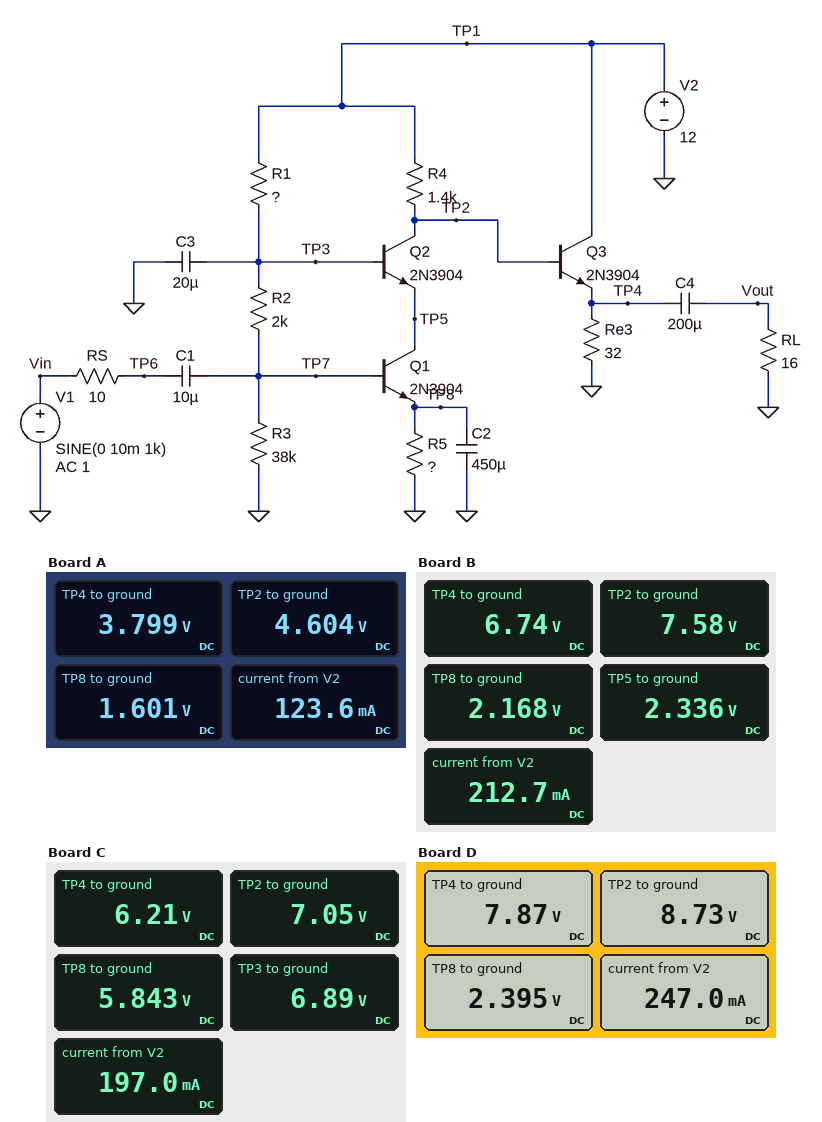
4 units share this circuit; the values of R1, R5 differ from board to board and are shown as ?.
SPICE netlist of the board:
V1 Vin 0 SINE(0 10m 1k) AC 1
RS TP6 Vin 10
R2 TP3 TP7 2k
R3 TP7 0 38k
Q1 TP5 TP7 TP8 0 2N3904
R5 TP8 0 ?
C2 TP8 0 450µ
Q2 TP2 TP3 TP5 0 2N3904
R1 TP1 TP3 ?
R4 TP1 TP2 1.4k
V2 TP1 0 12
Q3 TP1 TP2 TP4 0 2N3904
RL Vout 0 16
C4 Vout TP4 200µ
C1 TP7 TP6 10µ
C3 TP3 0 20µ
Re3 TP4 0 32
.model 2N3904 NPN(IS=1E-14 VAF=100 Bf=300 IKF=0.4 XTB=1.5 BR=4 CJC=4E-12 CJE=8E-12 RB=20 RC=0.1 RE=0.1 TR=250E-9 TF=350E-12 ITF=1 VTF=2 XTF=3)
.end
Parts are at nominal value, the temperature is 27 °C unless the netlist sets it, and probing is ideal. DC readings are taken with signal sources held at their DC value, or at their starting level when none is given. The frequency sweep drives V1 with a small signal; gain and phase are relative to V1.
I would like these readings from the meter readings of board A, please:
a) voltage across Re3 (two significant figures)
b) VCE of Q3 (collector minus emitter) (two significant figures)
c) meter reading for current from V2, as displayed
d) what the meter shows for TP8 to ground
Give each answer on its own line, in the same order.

3.8 V
8.2 V
123.6 mA
1.601 V
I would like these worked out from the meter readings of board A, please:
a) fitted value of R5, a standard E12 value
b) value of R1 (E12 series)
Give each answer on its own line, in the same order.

330 Ω
100 kΩ
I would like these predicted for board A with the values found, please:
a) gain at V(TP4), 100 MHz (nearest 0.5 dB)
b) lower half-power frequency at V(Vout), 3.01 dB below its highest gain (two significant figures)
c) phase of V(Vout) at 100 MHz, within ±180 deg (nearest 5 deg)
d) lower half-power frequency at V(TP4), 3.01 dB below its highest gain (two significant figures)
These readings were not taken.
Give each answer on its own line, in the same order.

1.0 dB
91 Hz
-35 deg
66 Hz
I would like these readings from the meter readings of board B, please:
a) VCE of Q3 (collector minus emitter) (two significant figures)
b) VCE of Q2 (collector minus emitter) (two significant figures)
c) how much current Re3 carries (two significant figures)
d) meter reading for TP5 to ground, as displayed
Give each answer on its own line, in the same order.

5.3 V
5.2 V
210 mA
2.336 V
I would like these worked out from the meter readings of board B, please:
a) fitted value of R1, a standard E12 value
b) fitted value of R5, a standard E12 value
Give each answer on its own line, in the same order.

100 kΩ
1 kΩ
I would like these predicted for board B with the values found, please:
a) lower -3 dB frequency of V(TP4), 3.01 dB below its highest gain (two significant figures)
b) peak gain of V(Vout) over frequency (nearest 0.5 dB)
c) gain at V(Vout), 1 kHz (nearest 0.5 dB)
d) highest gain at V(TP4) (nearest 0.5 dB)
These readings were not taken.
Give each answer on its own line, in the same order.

26 Hz
35.5 dB
35.5 dB
35.5 dB
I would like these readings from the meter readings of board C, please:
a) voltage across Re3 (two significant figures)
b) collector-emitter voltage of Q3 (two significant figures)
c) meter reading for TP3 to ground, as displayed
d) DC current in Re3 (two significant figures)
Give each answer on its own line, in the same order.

6.2 V
5.8 V
6.89 V
190 mA
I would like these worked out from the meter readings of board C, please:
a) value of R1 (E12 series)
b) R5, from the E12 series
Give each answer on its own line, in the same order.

27 kΩ
2.2 kΩ
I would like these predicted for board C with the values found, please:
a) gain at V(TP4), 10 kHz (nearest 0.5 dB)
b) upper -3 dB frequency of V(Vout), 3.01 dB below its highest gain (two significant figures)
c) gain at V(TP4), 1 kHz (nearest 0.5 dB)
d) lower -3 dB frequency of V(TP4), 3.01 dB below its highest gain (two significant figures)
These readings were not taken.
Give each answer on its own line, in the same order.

37.5 dB
4.9 MHz
37.5 dB
31 Hz
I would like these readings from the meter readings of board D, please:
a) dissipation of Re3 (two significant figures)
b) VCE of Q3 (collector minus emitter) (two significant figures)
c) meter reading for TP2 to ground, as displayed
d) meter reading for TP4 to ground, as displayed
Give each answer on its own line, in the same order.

1.9 W
4.1 V
8.73 V
7.87 V
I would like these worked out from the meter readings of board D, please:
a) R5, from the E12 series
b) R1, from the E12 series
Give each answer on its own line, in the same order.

2.2 kΩ
100 kΩ
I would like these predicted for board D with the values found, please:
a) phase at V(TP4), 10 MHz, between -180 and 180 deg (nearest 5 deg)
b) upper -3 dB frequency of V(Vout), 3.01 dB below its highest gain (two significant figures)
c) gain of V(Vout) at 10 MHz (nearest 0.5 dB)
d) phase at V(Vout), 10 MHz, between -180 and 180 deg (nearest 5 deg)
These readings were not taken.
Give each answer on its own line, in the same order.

105 deg
4.7 MHz
22.0 dB
105 deg
